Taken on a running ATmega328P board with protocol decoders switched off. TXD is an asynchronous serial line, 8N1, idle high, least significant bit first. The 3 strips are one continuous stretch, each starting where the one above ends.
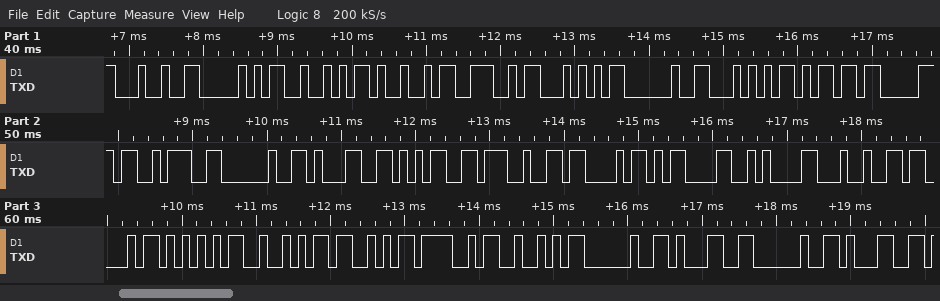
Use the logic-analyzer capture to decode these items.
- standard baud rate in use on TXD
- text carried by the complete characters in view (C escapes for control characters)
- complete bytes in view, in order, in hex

9600 baud
"$PRINT Tmp: 15'C\r\n$CURSOR 1 1"
24 50 52 49 4E 54 20 54 6D 70 3A 20 31 35 27 43 0D 0A 24 43 55 52 53 4F 52 20 31 20 31
